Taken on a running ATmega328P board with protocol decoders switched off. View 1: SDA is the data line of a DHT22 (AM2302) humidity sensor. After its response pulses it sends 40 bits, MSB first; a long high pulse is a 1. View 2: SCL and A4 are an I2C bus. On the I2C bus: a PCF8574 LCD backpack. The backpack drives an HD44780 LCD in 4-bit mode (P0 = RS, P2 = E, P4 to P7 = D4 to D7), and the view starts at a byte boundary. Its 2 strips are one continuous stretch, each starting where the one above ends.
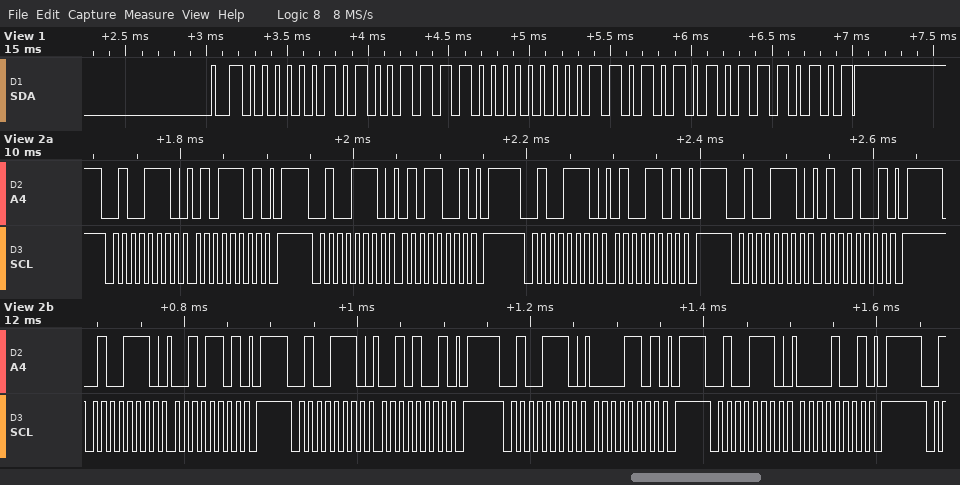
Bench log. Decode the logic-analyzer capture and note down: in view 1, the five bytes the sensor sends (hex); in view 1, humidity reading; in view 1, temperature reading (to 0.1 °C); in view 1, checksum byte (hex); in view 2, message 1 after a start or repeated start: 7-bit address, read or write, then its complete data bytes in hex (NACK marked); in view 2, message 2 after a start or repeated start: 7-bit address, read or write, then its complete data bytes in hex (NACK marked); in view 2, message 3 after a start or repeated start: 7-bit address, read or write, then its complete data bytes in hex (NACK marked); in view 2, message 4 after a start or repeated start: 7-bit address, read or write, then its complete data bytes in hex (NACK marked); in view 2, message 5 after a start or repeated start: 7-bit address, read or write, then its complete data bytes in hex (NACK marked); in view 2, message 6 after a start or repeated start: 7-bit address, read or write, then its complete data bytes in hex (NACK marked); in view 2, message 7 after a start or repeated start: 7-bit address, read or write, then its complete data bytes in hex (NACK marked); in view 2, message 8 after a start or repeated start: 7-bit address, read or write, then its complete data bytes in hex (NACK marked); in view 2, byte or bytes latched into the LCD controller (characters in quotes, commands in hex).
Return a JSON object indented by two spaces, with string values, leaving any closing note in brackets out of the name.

{
  "in view 1, the five bytes the sensor sends": "02 9E 00 D5 75",
  "in view 1, humidity reading": "67.0 %",
  "in view 1, temperature reading": "21.3 °C",
  "in view 1, checksum byte": "0x75",
  "in view 2, message 1 after a start or repeated start: 7-bit address, read or write, then its complete data bytes in hex": "0x27 write: 5D",
  "in view 2, message 2 after a start or repeated start: 7-bit address, read or write, then its complete data bytes in hex": "0x27 write: 59",
  "in view 2, message 3 after a start or repeated start: 7-bit address, read or write, then its complete data bytes in hex": "0x27 write: 4D",
  "in view 2, message 4 after a start or repeated start: 7-bit address, read or write, then its complete data bytes in hex": "0x27 write: 49",
  "in view 2, message 5 after a start or repeated start: 7-bit address, read or write, then its complete data bytes in hex": "0x27 write: 2D",
  "in view 2, message 6 after a start or repeated start: 7-bit address, read or write, then its complete data bytes in hex": "0x27 write: 29",
  "in view 2, message 7 after a start or repeated start: 7-bit address, read or write, then its complete data bytes in hex": "0x27 write: 0D",
  "in view 2, message 8 after a start or repeated start: 7-bit address, read or write, then its complete data bytes in hex": "0x27 write: 09",
  "in view 2, byte or bytes latched into the LCD controller": "'T' ' '"
}
